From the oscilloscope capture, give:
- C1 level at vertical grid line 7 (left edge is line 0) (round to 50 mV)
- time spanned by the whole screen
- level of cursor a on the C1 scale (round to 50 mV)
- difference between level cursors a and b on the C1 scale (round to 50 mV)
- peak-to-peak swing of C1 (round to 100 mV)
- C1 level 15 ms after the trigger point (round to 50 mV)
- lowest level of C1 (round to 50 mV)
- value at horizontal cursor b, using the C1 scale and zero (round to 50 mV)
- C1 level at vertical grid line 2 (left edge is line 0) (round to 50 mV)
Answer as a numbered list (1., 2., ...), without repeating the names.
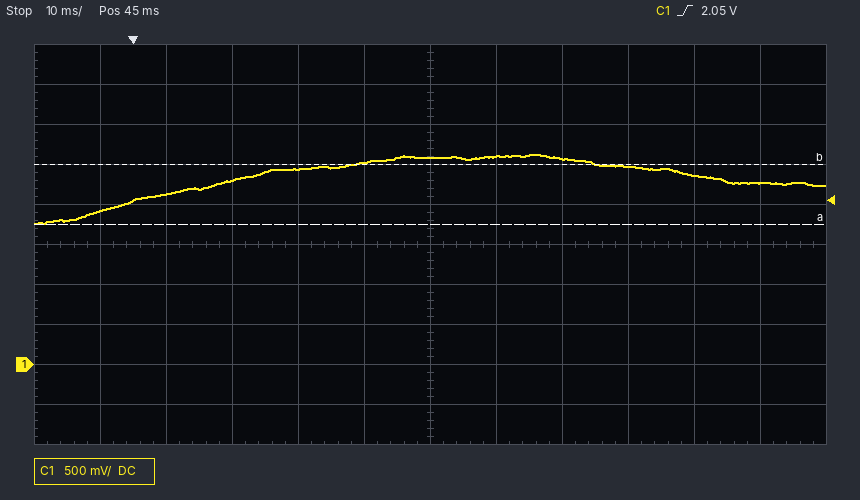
1. 2.60 V
2. 120 ms
3. 1.75 V
4. 750 mV
5. 900 mV
6. 2.30 V
7. 1.75 V
8. 2.50 V
9. 2.15 V
